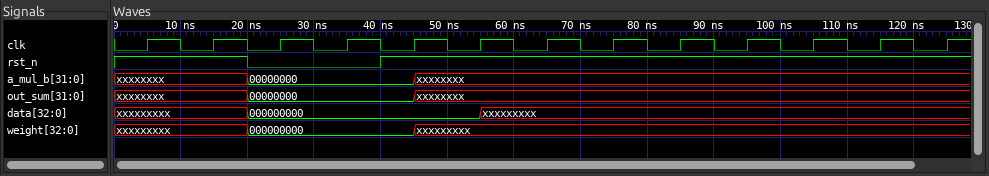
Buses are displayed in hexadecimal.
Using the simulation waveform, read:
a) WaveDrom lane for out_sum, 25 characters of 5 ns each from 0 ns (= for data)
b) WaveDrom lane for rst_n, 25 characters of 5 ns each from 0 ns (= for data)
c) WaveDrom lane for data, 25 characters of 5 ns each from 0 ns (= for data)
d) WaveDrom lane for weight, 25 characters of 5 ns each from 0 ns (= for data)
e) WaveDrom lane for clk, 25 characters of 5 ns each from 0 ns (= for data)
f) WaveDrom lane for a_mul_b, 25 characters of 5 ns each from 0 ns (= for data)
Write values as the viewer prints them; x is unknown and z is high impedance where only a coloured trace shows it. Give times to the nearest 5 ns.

{name: 'out_sum', wave: 'x...=....x...............', data: '00000000'}
{name: 'rst_n', wave: '1...0...1................'}
{name: 'data', wave: 'x...=......x.............', data: '000000000'}
{name: 'weight', wave: 'x...=....x...............', data: '000000000'}
{name: 'clk', wave: '0101010101010101010101010'}
{name: 'a_mul_b', wave: 'x...=....x...............', data: '00000000'}
